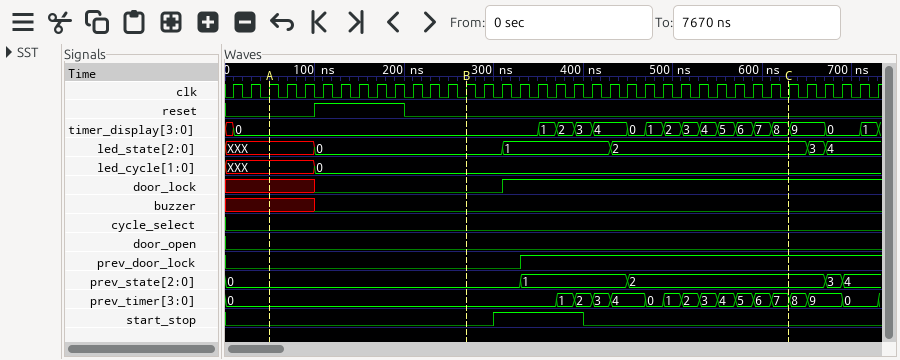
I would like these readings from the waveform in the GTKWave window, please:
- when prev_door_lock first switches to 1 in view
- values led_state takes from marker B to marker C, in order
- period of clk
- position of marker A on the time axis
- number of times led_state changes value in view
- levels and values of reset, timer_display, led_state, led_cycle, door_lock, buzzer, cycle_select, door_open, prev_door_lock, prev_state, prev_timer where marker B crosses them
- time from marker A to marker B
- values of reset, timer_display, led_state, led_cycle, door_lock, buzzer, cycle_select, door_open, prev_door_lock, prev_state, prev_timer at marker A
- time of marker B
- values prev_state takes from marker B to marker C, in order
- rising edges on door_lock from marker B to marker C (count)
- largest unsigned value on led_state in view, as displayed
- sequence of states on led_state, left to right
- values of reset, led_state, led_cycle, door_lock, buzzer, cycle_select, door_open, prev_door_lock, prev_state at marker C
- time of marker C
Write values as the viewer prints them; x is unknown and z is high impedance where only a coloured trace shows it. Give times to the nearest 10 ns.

330 ns
0, 1, 2
20 ns
50 ns
5
reset=0, timer_display=0, led_state=0, led_cycle=0, door_lock=0, buzzer=0, cycle_select=0, door_open=0, prev_door_lock=0, prev_state=0, prev_timer=0
220 ns
reset=0, timer_display=0, led_state=XXX, led_cycle=XXX, door_lock=x, buzzer=x, cycle_select=0, door_open=0, prev_door_lock=0, prev_state=0, prev_timer=0
270 ns
0, 1, 2
1
4
XXX, 0, 1, 2, 3, 4
reset=0, led_state=2, led_cycle=0, door_lock=1, buzzer=0, cycle_select=0, door_open=0, prev_door_lock=1, prev_state=2
630 ns
